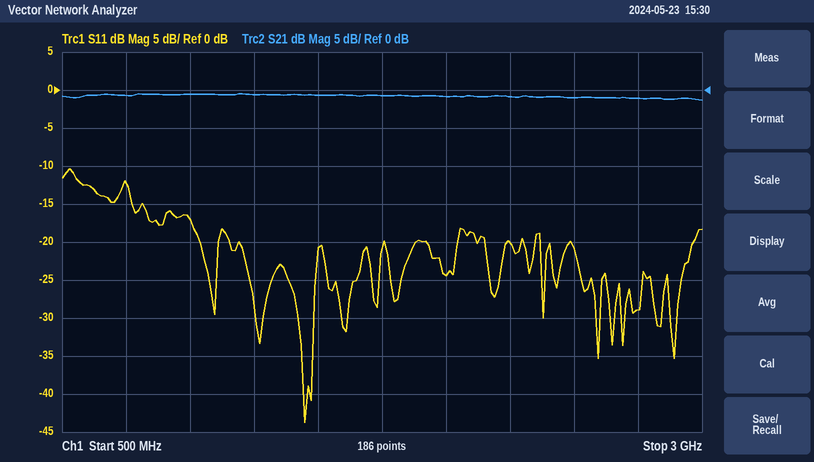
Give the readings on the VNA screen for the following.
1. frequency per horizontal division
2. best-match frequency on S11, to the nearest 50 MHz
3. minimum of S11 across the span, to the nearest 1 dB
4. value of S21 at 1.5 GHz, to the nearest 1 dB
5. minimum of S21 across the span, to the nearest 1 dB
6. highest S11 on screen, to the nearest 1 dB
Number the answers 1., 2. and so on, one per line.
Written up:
1. 250 MHz
2. 1.45 GHz
3. -44 dB
4. -1 dB
5. -1 dB
6. -10 dB
